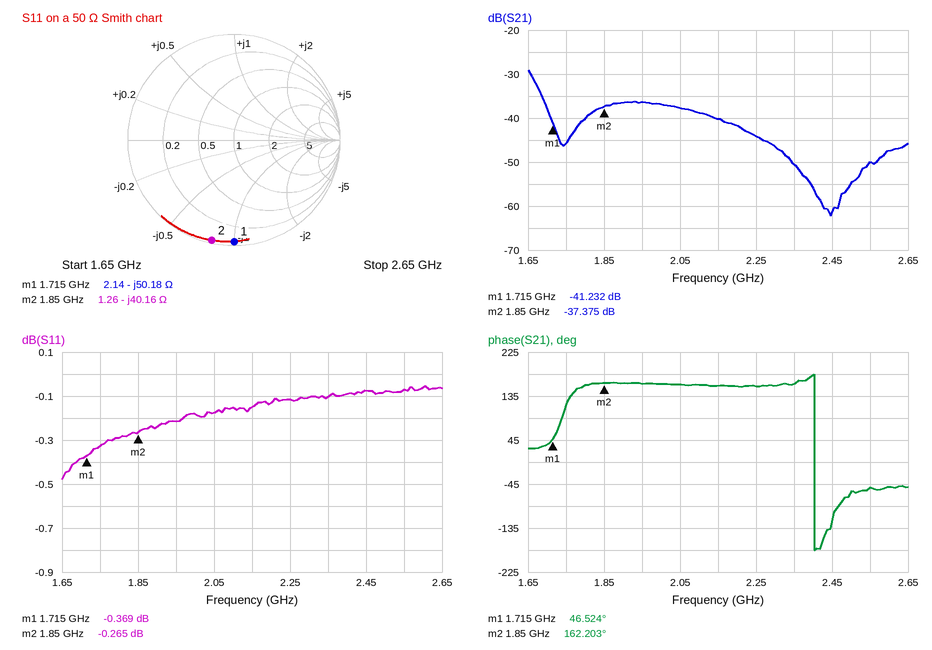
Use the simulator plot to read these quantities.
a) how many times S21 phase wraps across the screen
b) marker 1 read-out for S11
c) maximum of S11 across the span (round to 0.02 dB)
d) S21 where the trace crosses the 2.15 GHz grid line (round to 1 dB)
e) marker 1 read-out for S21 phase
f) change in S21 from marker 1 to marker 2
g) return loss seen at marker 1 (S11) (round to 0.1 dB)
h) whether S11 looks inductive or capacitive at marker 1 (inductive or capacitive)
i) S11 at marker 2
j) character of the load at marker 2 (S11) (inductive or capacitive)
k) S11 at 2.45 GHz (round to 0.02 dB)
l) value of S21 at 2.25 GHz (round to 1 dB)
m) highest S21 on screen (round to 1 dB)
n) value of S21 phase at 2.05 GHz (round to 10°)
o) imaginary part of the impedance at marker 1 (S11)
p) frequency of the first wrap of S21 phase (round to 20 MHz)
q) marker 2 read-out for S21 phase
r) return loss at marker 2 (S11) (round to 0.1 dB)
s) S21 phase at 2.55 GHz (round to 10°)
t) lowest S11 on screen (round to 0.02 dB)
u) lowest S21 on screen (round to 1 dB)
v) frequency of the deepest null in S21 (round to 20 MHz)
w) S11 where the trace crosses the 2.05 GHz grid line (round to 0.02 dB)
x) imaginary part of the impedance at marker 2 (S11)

1
-0.369 dB
-0.06 dB
-40 dB
46.524°
3.857 dB
0.4 dB
capacitive
-0.265 dB
capacitive
-0.08 dB
-44 dB
-29 dB
160°
-50.18 Ω
2.40 GHz
162.203°
0.3 dB
-50°
-0.48 dB
-62 dB
2.44 GHz
-0.18 dB
-40.16 Ω
